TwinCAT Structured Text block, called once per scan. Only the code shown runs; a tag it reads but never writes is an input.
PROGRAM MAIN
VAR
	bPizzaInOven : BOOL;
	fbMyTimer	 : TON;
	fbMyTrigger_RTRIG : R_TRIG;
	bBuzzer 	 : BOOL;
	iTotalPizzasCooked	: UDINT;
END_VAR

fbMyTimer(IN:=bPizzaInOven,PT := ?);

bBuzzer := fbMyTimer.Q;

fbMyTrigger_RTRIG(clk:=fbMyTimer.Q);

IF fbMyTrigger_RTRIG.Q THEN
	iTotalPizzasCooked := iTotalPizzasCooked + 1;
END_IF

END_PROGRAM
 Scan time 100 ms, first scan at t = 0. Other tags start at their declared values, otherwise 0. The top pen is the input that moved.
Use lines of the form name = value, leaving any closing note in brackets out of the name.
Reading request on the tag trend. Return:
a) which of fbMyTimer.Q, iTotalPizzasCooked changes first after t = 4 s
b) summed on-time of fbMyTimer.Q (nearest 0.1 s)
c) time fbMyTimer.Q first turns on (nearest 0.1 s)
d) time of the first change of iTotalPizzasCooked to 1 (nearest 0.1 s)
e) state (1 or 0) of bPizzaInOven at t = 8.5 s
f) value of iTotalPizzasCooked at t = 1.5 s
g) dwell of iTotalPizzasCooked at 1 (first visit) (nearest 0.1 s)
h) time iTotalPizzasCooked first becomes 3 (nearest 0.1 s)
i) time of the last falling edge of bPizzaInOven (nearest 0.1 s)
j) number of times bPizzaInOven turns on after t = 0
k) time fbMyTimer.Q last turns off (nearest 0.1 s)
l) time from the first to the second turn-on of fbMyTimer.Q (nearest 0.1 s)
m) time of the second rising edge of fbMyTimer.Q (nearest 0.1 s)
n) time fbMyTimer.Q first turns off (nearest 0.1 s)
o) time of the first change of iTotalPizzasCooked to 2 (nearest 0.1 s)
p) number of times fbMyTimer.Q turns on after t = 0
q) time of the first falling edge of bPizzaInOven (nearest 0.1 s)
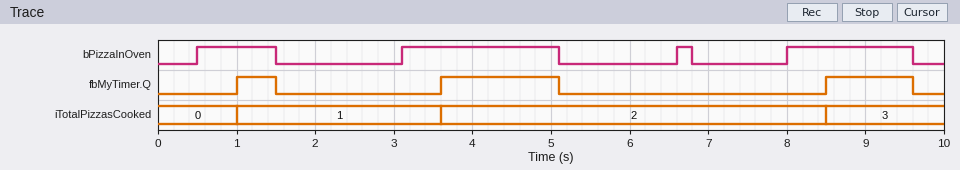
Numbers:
which of fbMyTimer.Q, iTotalPizzasCooked changes first after t = 4 s = fbMyTimer.Q
summed on-time of fbMyTimer.Q = 3.1 s
time fbMyTimer.Q first turns on = 1.0 s
time of the first change of iTotalPizzasCooked to 1 = 1.0 s
state (1 or 0) of bPizzaInOven at t = 8.5 s = 1
value of iTotalPizzasCooked at t = 1.5 s = 1
dwell of iTotalPizzasCooked at 1 (first visit) = 2.6 s
time iTotalPizzasCooked first becomes 3 = 8.5 s
time of the last falling edge of bPizzaInOven = 9.6 s
number of times bPizzaInOven turns on after t = 0 = 4
time fbMyTimer.Q last turns off = 9.6 s
time from the first to the second turn-on of fbMyTimer.Q = 2.6 s
time of the second rising edge of fbMyTimer.Q = 3.6 s
time fbMyTimer.Q first turns off = 1.5 s
time of the first change of iTotalPizzasCooked to 2 = 3.6 s
number of times fbMyTimer.Q turns on after t = 0 = 3
time of the first falling edge of bPizzaInOven = 1.5 s
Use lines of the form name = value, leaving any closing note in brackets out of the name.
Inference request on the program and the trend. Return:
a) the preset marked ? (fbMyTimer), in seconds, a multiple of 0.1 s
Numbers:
the preset marked ? (fbMyTimer), in seconds, a multiple of 0.1 s = 0.5 s
